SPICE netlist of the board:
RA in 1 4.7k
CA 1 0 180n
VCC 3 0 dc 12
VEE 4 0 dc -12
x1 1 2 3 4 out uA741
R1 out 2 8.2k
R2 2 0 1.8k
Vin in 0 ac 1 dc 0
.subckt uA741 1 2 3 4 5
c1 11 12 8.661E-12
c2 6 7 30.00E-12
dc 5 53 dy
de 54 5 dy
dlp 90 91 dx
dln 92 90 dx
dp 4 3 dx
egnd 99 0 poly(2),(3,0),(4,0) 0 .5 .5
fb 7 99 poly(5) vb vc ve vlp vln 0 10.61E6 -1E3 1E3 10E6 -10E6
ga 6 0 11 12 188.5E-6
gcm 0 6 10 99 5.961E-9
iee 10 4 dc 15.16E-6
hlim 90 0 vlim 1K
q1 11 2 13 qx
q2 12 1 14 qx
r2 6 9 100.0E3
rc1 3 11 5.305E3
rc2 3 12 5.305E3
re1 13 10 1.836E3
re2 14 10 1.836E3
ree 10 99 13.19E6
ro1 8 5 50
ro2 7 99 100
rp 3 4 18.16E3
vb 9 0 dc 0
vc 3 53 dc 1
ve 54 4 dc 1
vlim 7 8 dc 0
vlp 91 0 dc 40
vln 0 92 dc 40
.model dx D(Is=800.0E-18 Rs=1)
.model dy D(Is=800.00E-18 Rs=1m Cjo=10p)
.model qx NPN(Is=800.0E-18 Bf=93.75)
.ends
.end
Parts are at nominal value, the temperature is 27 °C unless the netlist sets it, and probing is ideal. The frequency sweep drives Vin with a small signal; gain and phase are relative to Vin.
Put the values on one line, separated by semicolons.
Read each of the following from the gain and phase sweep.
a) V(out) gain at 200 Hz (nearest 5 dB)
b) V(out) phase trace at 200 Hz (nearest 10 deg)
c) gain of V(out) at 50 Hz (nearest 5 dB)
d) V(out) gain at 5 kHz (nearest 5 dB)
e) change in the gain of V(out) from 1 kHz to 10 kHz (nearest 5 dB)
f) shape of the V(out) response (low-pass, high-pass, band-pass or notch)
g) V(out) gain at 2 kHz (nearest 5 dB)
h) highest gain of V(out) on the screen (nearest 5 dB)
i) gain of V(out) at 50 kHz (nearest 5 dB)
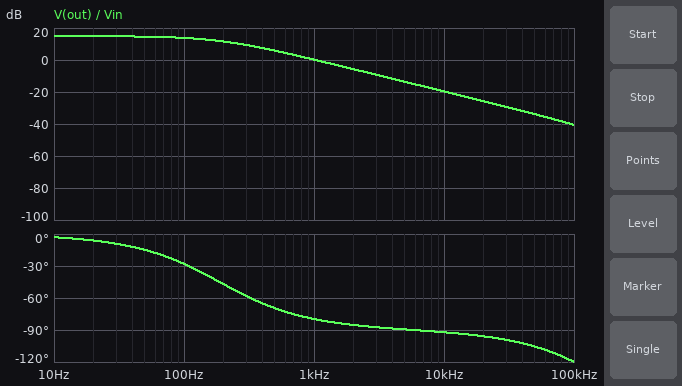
10 dB; -50 deg; 15 dB; -15 dB; -20 dB; low-pass; -5 dB; 15 dB; -35 dB
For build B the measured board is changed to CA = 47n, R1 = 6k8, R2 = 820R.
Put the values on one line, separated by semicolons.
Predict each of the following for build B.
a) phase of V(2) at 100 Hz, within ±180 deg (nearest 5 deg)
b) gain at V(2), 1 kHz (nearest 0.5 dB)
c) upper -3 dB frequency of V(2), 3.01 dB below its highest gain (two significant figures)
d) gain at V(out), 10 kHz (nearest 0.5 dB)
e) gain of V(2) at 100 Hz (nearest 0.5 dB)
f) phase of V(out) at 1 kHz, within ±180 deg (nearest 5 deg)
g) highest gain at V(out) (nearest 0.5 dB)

-10 deg; -4.5 dB; 720 Hz; -3.5 dB; 0 dB; -55 deg; 19.5 dB
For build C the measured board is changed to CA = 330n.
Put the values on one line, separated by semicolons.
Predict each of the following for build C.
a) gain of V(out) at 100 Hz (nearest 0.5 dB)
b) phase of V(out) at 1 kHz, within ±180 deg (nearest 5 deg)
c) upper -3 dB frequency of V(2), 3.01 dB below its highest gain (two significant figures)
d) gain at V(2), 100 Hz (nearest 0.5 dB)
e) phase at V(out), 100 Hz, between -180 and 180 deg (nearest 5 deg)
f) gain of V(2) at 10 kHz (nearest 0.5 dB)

12.0 dB; -85 deg; 100 Hz; -3.0 dB; -45 deg; -40.0 dB
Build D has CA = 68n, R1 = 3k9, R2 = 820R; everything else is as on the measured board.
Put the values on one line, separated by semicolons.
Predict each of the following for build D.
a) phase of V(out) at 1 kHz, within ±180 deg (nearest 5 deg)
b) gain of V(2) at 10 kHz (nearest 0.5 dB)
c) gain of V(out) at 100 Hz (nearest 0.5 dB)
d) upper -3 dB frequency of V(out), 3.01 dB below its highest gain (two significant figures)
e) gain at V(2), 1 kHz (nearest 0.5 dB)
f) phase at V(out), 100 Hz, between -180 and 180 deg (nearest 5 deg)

-65 deg; -26.0 dB; 15.0 dB; 500 Hz; -7.0 dB; -10 deg
